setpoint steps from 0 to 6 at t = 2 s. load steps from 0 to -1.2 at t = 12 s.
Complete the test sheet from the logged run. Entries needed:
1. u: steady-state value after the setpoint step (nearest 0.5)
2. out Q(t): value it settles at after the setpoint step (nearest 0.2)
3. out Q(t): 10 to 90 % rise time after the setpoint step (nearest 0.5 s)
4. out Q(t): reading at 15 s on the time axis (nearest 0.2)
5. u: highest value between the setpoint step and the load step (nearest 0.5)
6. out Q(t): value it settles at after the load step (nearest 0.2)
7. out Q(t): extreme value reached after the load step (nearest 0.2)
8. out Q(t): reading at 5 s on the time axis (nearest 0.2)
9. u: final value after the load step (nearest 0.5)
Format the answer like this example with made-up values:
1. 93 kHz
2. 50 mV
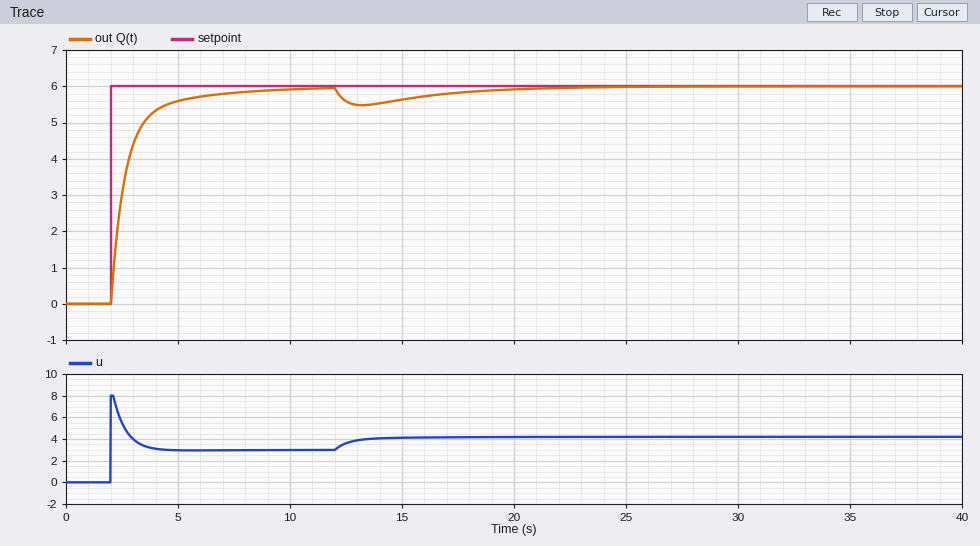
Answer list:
1. 3.0
2. 6.0
3. 2.0 s
4. 5.6
5. 8.0
6. 6.0
7. 5.4
8. 5.6
9. 4.0
